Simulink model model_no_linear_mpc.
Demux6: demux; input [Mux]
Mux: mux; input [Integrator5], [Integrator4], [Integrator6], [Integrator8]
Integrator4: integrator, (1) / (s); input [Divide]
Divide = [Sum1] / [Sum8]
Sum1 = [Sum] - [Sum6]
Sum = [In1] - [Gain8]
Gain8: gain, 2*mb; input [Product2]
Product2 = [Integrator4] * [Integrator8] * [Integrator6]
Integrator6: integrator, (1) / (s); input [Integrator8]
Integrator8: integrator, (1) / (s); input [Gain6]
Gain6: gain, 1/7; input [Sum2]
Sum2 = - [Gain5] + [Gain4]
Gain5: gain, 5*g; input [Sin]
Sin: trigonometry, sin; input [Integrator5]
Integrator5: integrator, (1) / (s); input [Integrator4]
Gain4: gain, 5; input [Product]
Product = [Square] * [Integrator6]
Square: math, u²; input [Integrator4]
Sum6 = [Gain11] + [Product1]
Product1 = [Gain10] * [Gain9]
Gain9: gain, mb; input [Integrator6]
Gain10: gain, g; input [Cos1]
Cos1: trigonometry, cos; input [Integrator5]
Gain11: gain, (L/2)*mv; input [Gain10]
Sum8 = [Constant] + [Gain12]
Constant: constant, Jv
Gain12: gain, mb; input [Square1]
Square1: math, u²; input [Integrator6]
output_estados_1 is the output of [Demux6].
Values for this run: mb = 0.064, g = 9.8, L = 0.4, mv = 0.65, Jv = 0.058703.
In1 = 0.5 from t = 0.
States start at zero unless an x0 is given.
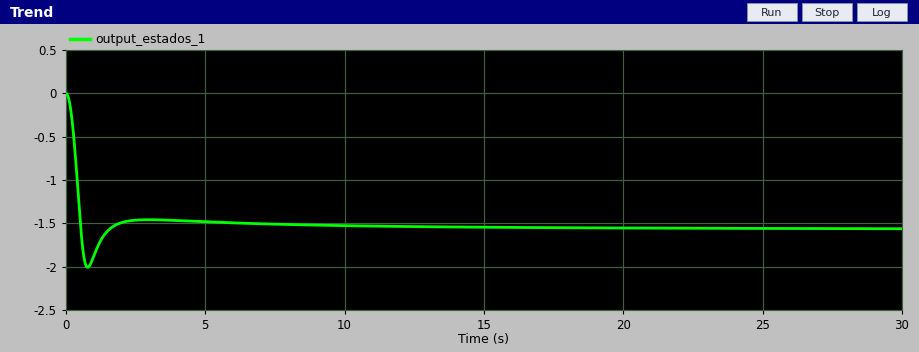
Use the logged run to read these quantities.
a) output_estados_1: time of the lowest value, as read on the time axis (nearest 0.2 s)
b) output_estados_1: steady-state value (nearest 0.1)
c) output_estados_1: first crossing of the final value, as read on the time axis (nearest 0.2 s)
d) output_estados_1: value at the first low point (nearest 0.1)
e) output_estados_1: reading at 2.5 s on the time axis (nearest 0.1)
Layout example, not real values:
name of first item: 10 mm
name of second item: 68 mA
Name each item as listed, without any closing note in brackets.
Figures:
output_estados_1: time of the lowest value, as read on the time axis: 0.8 s
output_estados_1: steady-state value: -1.6
output_estados_1: first crossing of the final value, as read on the time axis: 0.6 s
output_estados_1: value at the first low point: -2.0
output_estados_1: reading at 2.5 s on the time axis: -1.5
